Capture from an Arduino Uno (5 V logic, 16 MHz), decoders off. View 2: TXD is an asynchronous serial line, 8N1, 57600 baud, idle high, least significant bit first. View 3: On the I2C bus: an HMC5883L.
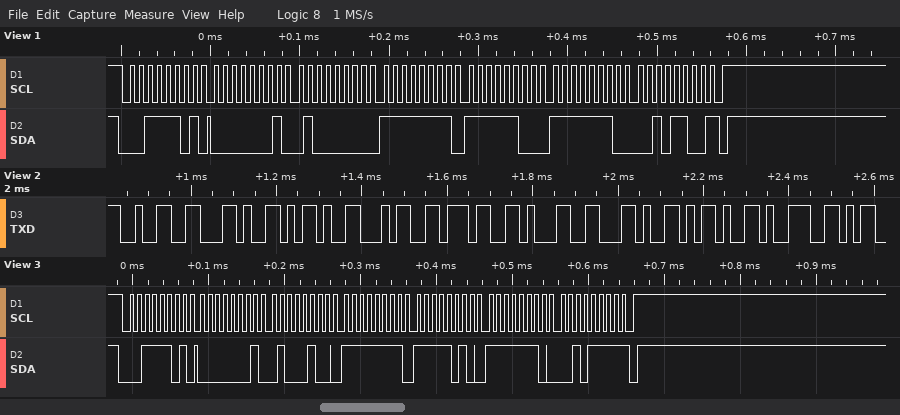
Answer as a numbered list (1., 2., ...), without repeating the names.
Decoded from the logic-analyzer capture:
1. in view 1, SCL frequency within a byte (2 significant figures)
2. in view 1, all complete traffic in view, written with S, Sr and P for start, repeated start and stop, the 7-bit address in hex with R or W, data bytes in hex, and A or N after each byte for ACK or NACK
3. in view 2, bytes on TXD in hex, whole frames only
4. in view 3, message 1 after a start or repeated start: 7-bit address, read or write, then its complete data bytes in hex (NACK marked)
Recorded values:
1. 100 kHz
2. S 1ER A 01 A 40 A FF A FC A FE A 2C N P
3. 0x32 0x2C 0x2D 0x34 0x37 0x31 0x2C 0x2D 0x39
4. 0x1E read: 01 44 FF FA FE 2F NACK
